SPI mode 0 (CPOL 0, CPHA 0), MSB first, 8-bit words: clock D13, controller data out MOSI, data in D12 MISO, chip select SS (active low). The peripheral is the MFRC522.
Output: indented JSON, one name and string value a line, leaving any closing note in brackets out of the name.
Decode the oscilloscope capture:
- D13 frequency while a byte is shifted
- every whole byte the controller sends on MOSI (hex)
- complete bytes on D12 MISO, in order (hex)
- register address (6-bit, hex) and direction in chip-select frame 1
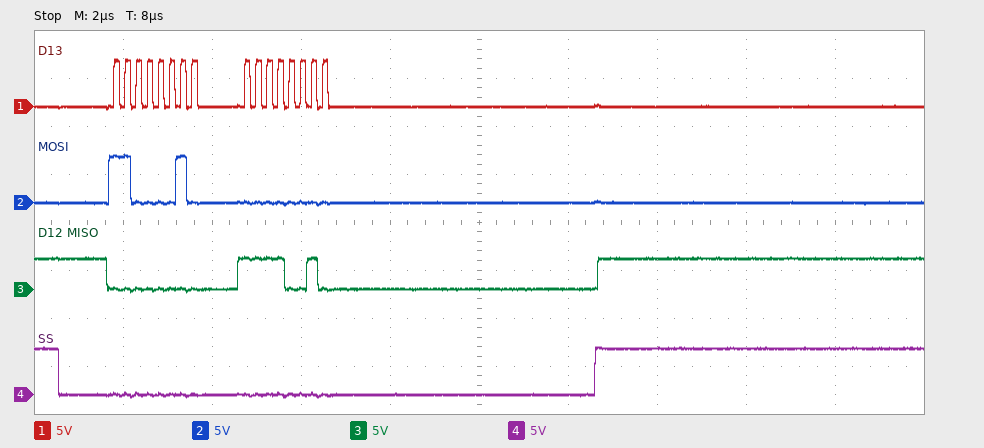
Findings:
{
  "D13 frequency while a byte is shifted": "4 MHz",
  "every whole byte the controller sends on MOSI": "C2 00",
  "complete bytes on D12 MISO, in order": "00 F2",
  "register address (6-bit, hex) and direction in chip-select frame 1": "0x21 read"
}
